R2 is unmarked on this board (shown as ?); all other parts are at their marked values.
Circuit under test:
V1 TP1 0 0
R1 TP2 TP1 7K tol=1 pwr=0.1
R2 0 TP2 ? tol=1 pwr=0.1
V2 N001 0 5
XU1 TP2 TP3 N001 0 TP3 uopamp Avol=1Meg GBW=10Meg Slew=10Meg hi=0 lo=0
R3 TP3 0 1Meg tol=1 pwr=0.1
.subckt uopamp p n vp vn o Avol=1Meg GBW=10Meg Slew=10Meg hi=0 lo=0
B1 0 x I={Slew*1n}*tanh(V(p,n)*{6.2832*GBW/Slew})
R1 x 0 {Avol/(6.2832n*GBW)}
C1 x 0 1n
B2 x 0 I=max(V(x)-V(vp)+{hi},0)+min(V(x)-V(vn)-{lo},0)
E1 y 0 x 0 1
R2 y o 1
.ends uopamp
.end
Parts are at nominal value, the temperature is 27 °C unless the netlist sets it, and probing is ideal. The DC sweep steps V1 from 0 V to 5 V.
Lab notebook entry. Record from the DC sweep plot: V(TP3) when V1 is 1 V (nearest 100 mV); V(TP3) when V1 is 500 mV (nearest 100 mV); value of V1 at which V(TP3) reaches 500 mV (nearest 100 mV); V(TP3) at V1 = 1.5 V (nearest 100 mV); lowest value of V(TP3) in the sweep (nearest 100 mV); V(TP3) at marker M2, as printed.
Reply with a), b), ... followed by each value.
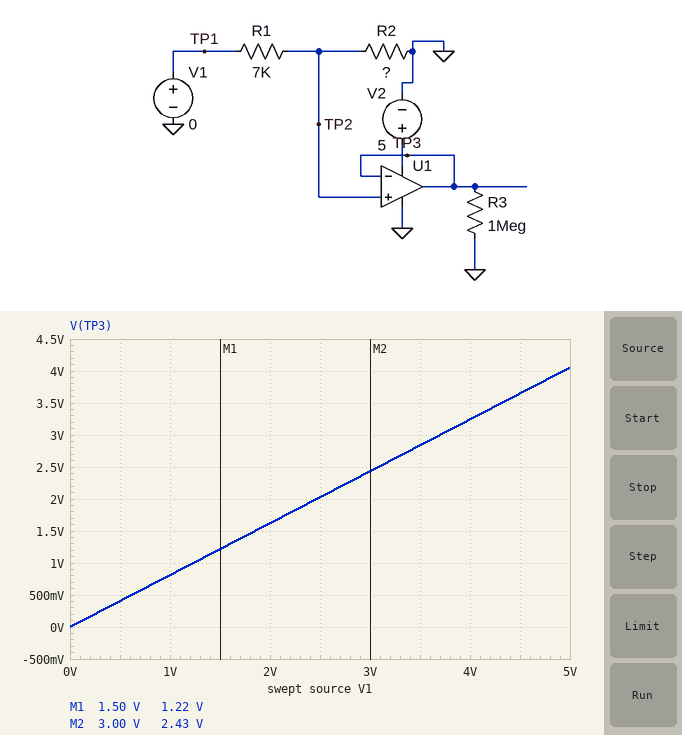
a) 800 mV
b) 400 mV
c) 600 mV
d) 1.2 V
e) 0 V
f) 2.43 V
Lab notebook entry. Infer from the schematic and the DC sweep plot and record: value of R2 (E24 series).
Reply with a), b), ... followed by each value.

a) 30 kΩ
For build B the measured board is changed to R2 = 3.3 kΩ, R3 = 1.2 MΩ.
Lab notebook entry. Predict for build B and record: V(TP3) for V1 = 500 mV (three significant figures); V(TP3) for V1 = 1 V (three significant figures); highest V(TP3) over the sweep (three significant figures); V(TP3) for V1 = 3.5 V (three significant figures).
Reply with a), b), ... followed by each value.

a) 160 mV
b) 320 mV
c) 1.60 V
d) 1.12 V
